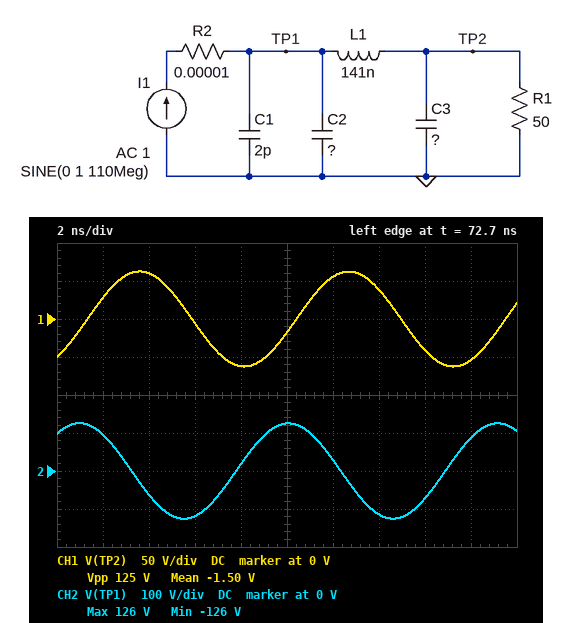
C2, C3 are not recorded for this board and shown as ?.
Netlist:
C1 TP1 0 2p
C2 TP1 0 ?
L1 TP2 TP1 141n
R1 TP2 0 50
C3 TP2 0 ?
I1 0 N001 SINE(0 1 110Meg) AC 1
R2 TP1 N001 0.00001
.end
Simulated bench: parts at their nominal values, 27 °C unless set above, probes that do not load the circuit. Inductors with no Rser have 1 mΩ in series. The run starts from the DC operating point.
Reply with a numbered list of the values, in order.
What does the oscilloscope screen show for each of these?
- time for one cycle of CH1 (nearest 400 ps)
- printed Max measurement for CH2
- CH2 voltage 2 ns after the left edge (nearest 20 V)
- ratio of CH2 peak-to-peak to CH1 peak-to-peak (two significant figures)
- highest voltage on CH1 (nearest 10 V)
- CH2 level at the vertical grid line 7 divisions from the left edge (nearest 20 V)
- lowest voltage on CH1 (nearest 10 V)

1. 9.2 ns
2. 126 V
3. 100 V
4. 2.0
5. 60 V
6. -120 V
7. -60 V
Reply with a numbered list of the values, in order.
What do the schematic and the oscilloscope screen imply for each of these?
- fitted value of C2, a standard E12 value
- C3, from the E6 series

1. 5.6 pF
2. 22 pF
